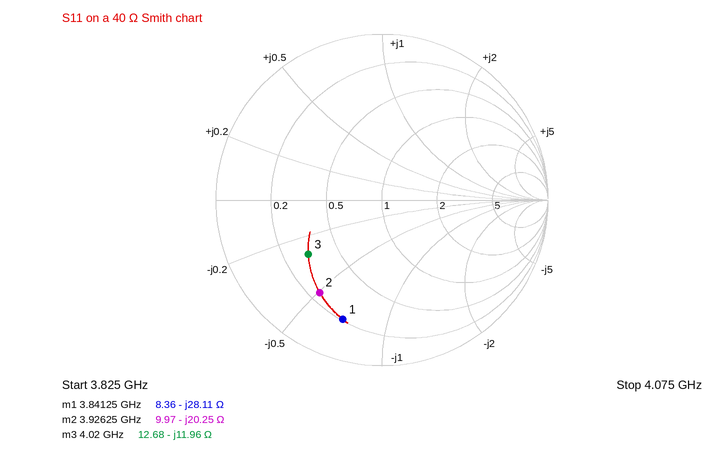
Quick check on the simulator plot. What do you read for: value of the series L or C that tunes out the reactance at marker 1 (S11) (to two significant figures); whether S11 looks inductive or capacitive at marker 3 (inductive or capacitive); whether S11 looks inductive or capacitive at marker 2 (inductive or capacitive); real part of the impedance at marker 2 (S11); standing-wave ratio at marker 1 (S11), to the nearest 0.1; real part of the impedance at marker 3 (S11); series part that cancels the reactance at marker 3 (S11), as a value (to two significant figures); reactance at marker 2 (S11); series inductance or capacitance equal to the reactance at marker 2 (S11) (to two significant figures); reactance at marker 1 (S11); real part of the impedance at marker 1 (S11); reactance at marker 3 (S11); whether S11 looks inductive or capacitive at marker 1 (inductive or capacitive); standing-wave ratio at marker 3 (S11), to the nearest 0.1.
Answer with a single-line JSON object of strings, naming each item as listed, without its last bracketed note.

{"value of the series L or C that tunes out the reactance at marker 1 (S11)": "1.2 nH", "whether S11 looks inductive or capacitive at marker 3": "capacitive", "whether S11 looks inductive or capacitive at marker 2": "capacitive", "real part of the impedance at marker 2": "9.97 Ω", "standing-wave ratio at marker 1 (S11), to the nearest 0.1": "7.2", "real part of the impedance at marker 3": "12.68 Ω", "series part that cancels the reactance at marker 3 (S11), as a value": "470 pH", "reactance at marker 2": "-20.25 Ω", "series inductance or capacitance equal to the reactance at marker 2 (S11)": "2.0 pF", "reactance at marker 1": "-28.11 Ω", "real part of the impedance at marker 1": "8.36 Ω", "reactance at marker 3": "-11.96 Ω", "whether S11 looks inductive or capacitive at marker 1": "capacitive", "standing-wave ratio at marker 3 (S11), to the nearest 0.1": "3.5"}
